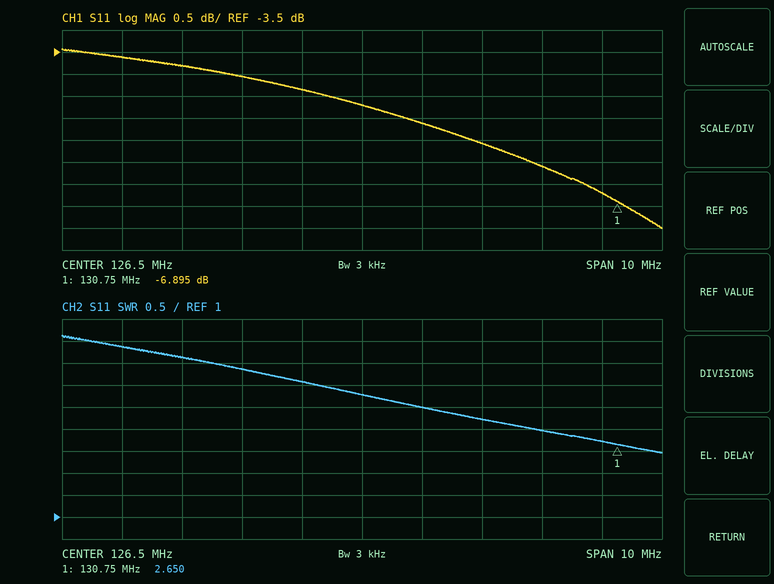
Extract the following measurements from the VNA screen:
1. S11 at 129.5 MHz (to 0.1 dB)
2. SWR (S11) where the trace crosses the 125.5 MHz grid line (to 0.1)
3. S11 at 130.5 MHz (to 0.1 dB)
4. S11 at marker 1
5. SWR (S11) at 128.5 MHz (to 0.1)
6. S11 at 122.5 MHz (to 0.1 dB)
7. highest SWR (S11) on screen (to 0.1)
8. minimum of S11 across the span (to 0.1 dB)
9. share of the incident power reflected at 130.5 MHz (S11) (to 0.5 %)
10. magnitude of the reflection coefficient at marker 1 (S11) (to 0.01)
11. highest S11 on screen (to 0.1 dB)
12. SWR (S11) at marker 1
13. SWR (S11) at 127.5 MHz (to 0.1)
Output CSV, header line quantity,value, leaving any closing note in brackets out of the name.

quantity,value
S11 at 129.5 MHz,-6.1 dB
SWR (S11) where the trace crosses the 125.5 MHz grid line,4.1
S11 at 130.5 MHz,-6.7 dB
S11 at marker 1,-6.895 dB
SWR (S11) at 128.5 MHz,3.2
S11 at 122.5 MHz,-3.6 dB
highest SWR (S11) on screen,5.1
minimum of S11 across the span,-7.5 dB
share of the incident power reflected at 130.5 MHz (S11),21.5 %
magnitude of the reflection coefficient at marker 1 (S11),0.45
highest S11 on screen,-3.4 dB
SWR (S11) at marker 1,2.650
SWR (S11) at 127.5 MHz,3.5
